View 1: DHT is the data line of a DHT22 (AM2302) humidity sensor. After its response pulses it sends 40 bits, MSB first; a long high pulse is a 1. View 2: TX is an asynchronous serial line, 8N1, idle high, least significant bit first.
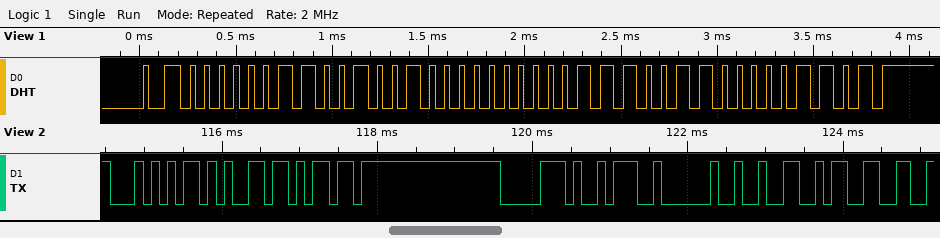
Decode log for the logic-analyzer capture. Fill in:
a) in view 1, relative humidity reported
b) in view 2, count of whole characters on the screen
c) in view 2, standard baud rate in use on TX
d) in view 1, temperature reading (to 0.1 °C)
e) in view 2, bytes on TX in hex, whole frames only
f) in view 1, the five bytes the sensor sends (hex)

80.4 %
8
9600 baud
23.0 °C
54 65 6D 70 3A 20 32 33
03 24 00 E6 0D
